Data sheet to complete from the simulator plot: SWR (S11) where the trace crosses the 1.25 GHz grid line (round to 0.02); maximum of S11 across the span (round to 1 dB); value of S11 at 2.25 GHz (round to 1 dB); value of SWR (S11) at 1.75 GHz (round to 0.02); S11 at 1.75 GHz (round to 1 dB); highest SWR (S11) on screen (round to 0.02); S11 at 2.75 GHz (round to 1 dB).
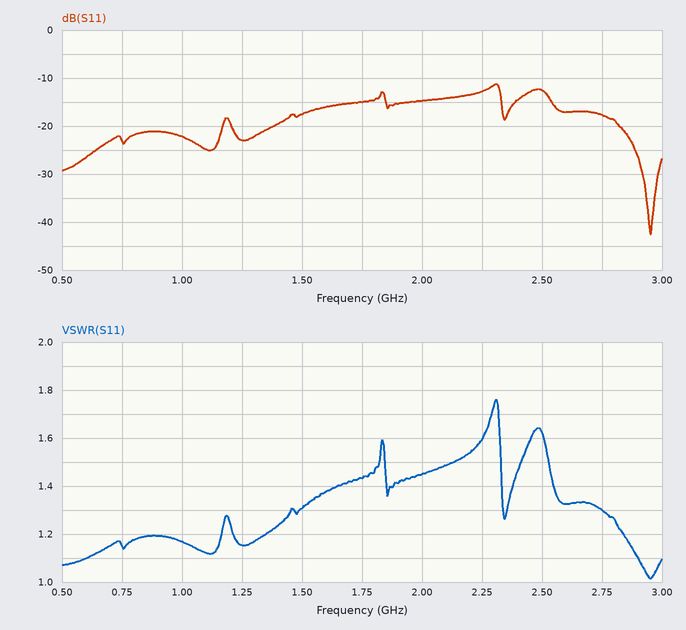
1.16
-11 dB
-13 dB
1.44
-15 dB
1.76
-18 dB
